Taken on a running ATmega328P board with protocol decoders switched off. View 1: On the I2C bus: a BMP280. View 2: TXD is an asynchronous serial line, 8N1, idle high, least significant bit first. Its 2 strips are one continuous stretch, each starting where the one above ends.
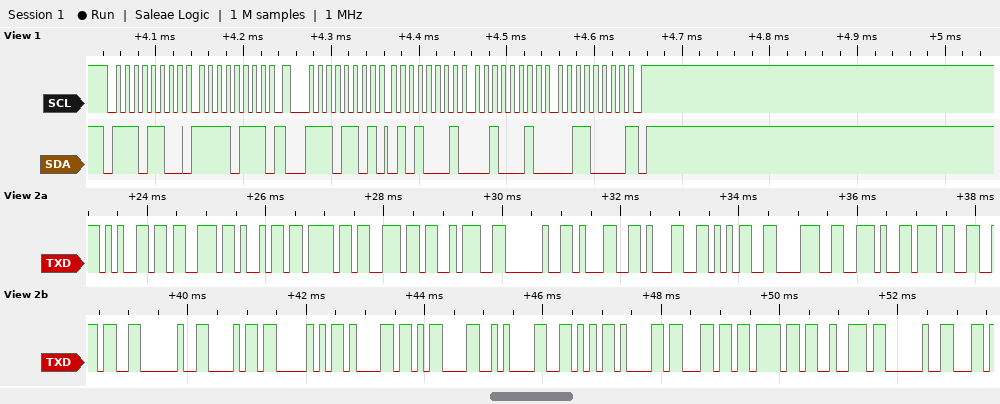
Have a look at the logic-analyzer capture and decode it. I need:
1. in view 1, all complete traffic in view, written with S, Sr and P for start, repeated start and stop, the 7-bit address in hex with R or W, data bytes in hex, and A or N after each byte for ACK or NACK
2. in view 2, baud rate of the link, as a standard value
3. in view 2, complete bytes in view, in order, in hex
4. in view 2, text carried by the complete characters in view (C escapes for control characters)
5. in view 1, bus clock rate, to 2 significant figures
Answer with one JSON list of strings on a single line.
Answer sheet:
["S 76W A F7 A Sr 76R A 51 A 22 A 30 N P", "9600 baud", "0x65 0x73 0x69 0x6F 0x6E 0x3A 0x20 0x31 0x31 0x35 0x38 0x2E 0x37 0x36 0x20 0x68 0x50 0x61 0x0D 0x0A 0x56 0x61 0x6C 0x6F 0x72 0x20", "\"esion: 1158.76 hPa\\r\\nValor \"", "100 kHz"]
